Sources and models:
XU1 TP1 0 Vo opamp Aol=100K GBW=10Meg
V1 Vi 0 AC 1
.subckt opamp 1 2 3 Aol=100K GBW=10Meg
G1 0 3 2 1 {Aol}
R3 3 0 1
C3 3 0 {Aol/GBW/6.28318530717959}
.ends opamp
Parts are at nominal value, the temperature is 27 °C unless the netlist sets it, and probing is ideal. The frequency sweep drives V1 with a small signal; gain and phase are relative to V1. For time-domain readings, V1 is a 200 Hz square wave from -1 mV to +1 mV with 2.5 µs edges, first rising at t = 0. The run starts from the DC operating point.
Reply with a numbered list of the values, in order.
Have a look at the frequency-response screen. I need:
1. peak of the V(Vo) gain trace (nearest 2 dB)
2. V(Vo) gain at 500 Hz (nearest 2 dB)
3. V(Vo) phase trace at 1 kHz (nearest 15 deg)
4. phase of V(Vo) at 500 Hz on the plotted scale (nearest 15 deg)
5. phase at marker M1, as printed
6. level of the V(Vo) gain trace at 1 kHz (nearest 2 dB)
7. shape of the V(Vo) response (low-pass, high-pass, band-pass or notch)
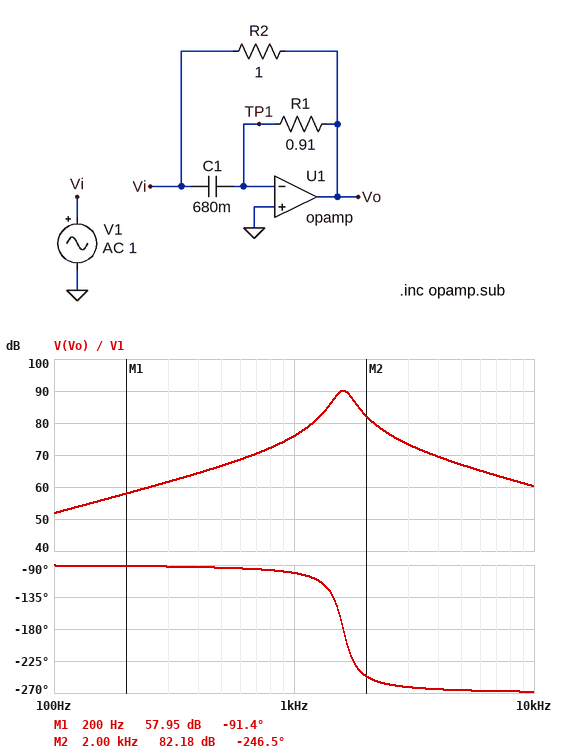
1. 90 dB
2. 66 dB
3. -105 deg
4. -90 deg
5. -91.4 deg
6. 76 dB
7. band-pass
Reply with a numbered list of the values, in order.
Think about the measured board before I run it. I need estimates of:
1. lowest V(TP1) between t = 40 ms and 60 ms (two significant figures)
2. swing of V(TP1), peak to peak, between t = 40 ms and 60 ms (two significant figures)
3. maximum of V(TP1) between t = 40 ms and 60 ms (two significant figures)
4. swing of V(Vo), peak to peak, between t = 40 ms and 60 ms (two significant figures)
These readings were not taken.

1. -1.8 mV
2. 3.7 mV
3. 1.8 mV
4. 20 V
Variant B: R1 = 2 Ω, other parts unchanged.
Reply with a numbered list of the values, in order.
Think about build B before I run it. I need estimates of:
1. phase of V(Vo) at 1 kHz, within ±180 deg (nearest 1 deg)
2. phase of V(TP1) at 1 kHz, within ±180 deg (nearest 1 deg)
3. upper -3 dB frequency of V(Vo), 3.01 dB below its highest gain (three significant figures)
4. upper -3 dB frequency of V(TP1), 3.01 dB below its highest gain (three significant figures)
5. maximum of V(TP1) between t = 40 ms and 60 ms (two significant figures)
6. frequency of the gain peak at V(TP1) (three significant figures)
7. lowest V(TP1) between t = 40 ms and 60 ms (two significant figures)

1. -146 deg
2. 110 deg
3. 1.21 kHz
4. 1.25 kHz
5. 2.1 mV
6. 1.10 kHz
7. -2.1 mV
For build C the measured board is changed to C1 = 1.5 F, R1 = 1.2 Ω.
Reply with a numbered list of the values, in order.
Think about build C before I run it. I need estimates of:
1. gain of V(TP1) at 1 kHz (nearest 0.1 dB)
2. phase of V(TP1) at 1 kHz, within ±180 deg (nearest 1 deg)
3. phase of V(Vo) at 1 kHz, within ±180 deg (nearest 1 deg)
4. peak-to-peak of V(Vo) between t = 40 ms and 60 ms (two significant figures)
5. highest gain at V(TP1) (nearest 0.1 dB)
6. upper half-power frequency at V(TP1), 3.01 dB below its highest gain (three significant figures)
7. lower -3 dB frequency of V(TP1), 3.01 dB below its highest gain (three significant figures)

1. 10.6 dB
2. 52 deg
3. 158 deg
4. 35 V
5. 10.9 dB
6. 1.15 kHz
7. 838 Hz
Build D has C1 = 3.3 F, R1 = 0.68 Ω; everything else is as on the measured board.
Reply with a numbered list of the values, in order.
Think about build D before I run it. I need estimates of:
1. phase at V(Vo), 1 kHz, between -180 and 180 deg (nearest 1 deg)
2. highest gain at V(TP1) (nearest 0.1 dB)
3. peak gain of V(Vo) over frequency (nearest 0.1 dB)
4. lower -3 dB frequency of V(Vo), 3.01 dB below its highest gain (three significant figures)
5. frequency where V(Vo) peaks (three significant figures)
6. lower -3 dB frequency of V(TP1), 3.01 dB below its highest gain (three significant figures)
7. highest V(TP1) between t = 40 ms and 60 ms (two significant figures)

1. 140 deg
2. 8.5 dB
3. 89.2 dB
4. 686 Hz
5. 842 Hz
6. 727 Hz
7. 1.9 mV
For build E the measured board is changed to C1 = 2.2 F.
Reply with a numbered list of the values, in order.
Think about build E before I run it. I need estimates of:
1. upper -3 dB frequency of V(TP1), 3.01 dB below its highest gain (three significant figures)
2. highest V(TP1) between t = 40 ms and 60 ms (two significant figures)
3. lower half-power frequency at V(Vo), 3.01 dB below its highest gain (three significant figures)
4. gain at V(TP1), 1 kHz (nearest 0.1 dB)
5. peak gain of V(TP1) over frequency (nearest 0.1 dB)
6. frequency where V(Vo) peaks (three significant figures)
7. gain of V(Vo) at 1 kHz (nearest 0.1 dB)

1. 1.14 kHz
2. 1.9 mV
3. 750 Hz
4. 9.0 dB
5. 9.8 dB
6. 892 Hz
7. 88.6 dB
